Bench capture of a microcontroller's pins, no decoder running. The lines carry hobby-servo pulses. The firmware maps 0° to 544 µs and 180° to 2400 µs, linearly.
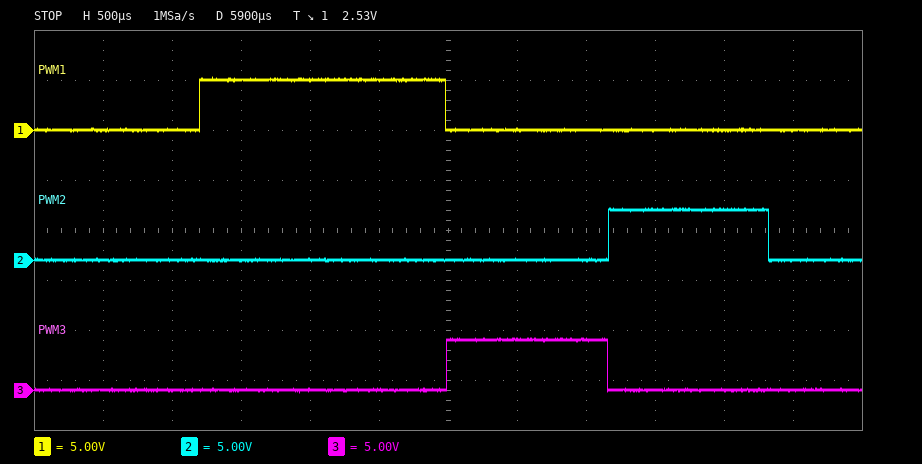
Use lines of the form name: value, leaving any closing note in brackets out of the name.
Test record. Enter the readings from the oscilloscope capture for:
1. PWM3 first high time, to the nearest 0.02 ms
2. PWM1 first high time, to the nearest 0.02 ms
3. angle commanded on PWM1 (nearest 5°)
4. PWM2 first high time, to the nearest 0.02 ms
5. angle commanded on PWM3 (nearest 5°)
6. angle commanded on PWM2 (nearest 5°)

PWM3 first high time, to the nearest 0.02 ms: 1.16 ms
PWM1 first high time, to the nearest 0.02 ms: 1.78 ms
angle commanded on PWM1: 120°
PWM2 first high time, to the nearest 0.02 ms: 1.16 ms
angle commanded on PWM3: 60°
angle commanded on PWM2: 60°
